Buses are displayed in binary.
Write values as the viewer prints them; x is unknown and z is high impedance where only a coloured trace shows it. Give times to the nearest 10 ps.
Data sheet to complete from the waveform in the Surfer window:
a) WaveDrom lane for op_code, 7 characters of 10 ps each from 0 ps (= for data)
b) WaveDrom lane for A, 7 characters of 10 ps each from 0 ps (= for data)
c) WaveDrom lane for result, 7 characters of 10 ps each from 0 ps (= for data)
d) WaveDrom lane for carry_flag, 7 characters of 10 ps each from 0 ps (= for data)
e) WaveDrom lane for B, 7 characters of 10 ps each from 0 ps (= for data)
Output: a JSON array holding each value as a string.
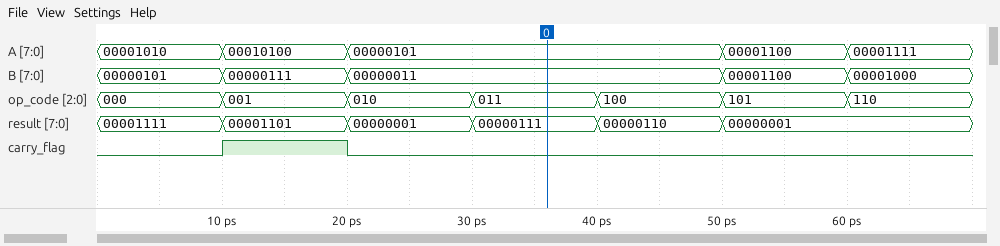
["{name: 'op_code', wave: '=======', data: '000 001 010 011 100 101 110'}", "{name: 'A', wave: '===..==', data: '00001010 00010100 00000101 00001100 00001111'}", "{name: 'result', wave: '======.', data: '00001111 00001101 00000001 00000111 00000110 00000001'}", "{name: 'carry_flag', wave: '010....'}", "{name: 'B', wave: '===..==', data: '00000101 00000111 00000011 00001100 00001000'}"]
